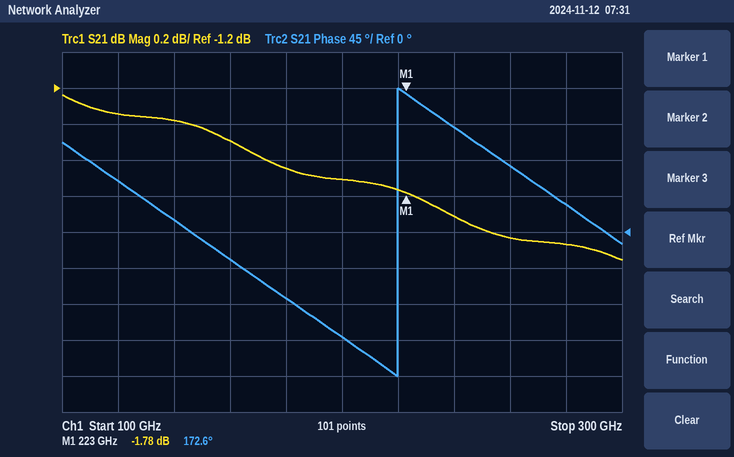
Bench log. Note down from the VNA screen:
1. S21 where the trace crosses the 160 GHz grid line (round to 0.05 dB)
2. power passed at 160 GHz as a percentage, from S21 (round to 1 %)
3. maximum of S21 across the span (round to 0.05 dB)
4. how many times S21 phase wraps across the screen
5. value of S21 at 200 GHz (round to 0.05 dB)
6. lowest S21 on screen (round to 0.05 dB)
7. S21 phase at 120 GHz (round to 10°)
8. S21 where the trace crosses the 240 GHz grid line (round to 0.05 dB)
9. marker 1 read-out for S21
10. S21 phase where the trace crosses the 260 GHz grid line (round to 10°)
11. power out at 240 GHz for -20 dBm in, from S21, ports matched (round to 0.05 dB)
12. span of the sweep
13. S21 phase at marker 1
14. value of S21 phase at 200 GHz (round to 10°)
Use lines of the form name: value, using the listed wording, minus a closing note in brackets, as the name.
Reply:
S21 where the trace crosses the 160 GHz grid line: -1.50 dB
power passed at 160 GHz as a percentage, from S21: 71 %
maximum of S21 across the span: -1.25 dB
how many times S21 phase wraps across the screen: 1
value of S21 at 200 GHz: -1.70 dB
lowest S21 on screen: -2.15 dB
S21 phase at 120 GHz: 60°
S21 where the trace crosses the 240 GHz grid line: -1.90 dB
marker 1 read-out for S21: -1.78 dB
S21 phase where the trace crosses the 260 GHz grid line: 80°
power out at 240 GHz for -20 dBm in, from S21, ports matched: -21.90 dBm
span of the sweep: 200 GHz
S21 phase at marker 1: 172.6°
value of S21 phase at 200 GHz: -130°
